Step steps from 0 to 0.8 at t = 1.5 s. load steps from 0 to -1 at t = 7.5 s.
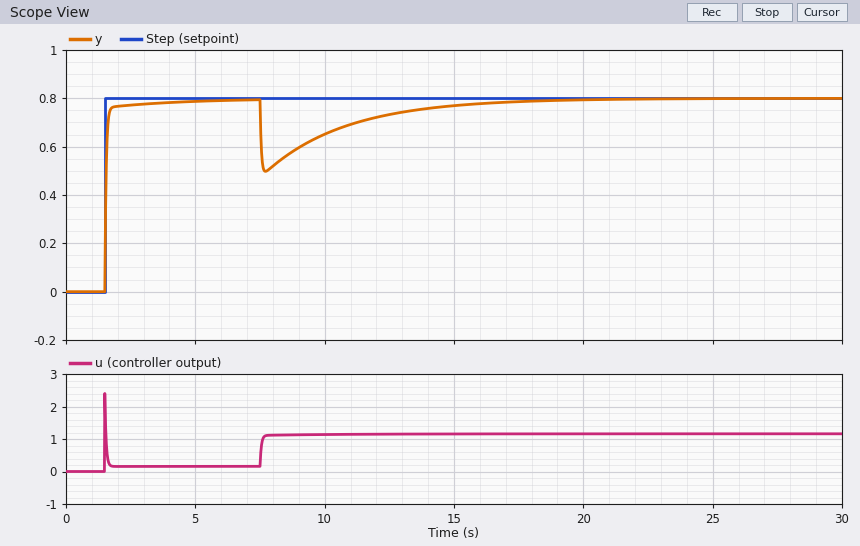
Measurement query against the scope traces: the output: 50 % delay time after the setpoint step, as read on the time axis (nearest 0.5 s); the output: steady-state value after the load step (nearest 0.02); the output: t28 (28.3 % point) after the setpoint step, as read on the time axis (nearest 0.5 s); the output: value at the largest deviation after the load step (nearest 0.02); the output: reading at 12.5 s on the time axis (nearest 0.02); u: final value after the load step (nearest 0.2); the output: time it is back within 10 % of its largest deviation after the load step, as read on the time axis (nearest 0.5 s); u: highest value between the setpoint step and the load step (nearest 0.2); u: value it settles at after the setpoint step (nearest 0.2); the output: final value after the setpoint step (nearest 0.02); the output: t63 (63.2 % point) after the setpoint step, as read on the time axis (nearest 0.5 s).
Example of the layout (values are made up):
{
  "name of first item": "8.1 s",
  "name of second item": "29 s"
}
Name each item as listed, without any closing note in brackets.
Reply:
{
  "the output: 50 % delay time after the setpoint step, as read on the time axis": "1.5 s",
  "the output: steady-state value after the load step": "0.80",
  "the output: t28 (28.3 % point) after the setpoint step, as read on the time axis": "1.5 s",
  "the output: value at the largest deviation after the load step": "0.50",
  "the output: reading at 12.5 s on the time axis": "0.74",
  "u: final value after the load step": "1.2",
  "the output: time it is back within 10 % of its largest deviation after the load step, as read on the time axis": "15.0 s",
  "u: highest value between the setpoint step and the load step": "2.4",
  "u: value it settles at after the setpoint step": "0.2",
  "the output: final value after the setpoint step": "0.80",
  "the output: t63 (63.2 % point) after the setpoint step, as read on the time axis": "1.5 s"
}
